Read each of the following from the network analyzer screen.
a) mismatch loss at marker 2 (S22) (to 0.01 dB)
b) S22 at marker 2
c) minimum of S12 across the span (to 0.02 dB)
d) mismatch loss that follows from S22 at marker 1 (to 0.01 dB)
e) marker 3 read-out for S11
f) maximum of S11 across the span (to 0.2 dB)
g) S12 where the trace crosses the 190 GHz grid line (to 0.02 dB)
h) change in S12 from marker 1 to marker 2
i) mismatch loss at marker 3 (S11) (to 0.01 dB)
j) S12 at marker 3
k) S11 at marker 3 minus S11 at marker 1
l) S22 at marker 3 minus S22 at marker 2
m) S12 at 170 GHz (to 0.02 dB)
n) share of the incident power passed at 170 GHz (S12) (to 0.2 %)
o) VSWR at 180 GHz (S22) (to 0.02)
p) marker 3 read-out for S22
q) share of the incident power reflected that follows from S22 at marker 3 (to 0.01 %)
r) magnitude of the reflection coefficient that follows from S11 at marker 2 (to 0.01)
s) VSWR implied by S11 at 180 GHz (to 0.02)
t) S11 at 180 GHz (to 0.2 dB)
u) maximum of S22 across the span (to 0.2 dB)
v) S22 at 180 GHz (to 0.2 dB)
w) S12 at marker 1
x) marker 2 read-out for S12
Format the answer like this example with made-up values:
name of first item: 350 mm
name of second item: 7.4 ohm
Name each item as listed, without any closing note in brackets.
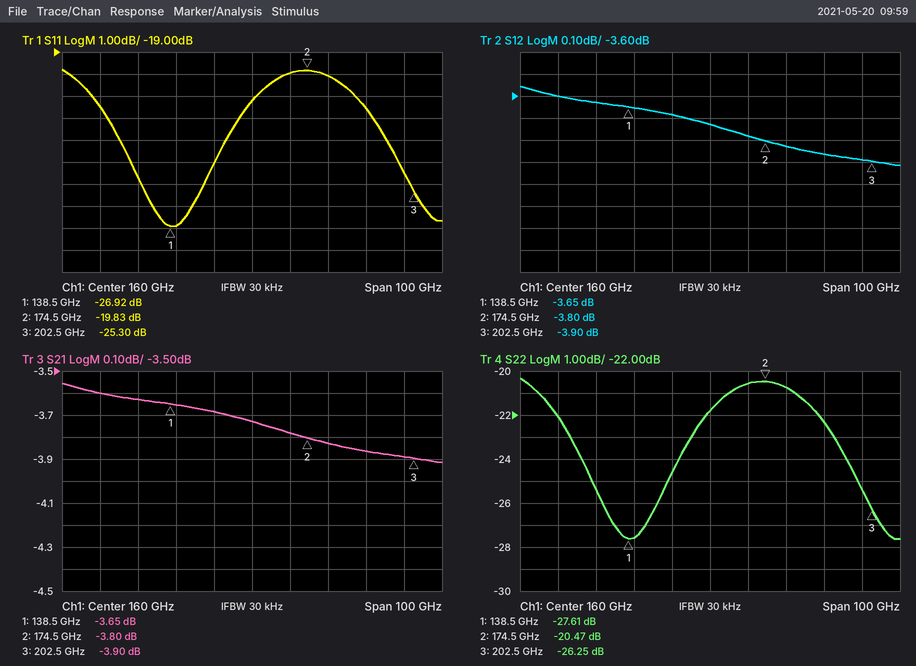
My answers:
mismatch loss at marker 2 (S22): 0.04 dB
S22 at marker 2: -20.47 dB
minimum of S12 across the span: -3.92 dB
mismatch loss that follows from S22 at marker 1: 0.01 dB
marker 3 read-out for S11: -25.30 dB
maximum of S11 across the span: -19.8 dB
S12 where the trace crosses the 190 GHz grid line: -3.86 dB
change in S12 from marker 1 to marker 2: -0.15 dB
mismatch loss at marker 3 (S11): 0.01 dB
S12 at marker 3: -3.90 dB
S11 at marker 3 minus S11 at marker 1: 1.62 dB
S22 at marker 3 minus S22 at marker 2: -5.78 dB
S12 at 170 GHz: -3.78 dB
share of the incident power passed at 170 GHz (S12): 41.8 %
VSWR at 180 GHz (S22): 1.20
marker 3 read-out for S22: -26.25 dB
share of the incident power reflected that follows from S22 at marker 3: 0.24 %
magnitude of the reflection coefficient that follows from S11 at marker 2: 0.10
VSWR implied by S11 at 180 GHz: 1.22
S11 at 180 GHz: -20.0 dB
maximum of S22 across the span: -20.4 dB
S22 at 180 GHz: -20.8 dB
S12 at marker 1: -3.65 dB
marker 2 read-out for S12: -3.80 dB
